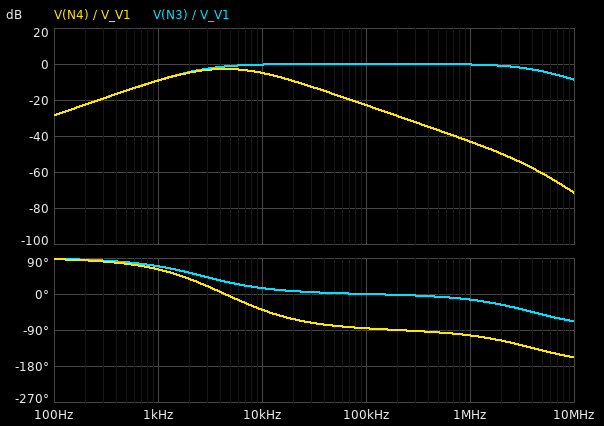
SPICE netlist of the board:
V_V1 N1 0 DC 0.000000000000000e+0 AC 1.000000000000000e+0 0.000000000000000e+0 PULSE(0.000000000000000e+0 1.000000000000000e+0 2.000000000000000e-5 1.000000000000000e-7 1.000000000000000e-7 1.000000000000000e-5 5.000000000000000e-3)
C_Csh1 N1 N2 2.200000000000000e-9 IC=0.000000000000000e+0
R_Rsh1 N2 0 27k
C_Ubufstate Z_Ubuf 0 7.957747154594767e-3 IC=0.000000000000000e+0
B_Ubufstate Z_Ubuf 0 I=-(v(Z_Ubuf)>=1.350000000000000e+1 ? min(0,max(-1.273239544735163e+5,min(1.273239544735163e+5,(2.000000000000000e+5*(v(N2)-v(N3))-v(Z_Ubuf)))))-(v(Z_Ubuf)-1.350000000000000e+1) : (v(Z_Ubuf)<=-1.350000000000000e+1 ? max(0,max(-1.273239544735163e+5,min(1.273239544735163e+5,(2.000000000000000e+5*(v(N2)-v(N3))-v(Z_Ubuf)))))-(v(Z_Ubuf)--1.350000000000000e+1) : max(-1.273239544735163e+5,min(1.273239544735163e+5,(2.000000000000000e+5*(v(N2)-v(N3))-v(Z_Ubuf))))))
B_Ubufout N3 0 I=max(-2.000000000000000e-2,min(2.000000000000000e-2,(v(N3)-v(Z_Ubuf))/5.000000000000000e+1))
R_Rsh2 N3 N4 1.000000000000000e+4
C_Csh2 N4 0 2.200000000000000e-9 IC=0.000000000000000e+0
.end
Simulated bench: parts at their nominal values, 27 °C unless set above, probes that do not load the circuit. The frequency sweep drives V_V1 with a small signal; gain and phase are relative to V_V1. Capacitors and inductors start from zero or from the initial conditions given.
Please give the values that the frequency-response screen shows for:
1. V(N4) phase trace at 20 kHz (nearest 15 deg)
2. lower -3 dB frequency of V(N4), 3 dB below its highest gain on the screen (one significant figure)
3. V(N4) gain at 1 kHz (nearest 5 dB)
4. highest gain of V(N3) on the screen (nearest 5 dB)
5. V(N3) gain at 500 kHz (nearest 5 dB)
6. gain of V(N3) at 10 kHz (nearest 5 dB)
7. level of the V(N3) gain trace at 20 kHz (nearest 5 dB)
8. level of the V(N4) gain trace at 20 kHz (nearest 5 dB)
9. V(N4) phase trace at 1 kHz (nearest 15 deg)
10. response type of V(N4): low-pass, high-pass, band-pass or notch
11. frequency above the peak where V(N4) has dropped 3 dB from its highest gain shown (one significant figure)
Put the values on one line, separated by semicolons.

-60 deg; 2 kHz; -10 dB; 0 dB; 0 dB; 0 dB; 0 dB; -10 dB; 60 deg; band-pass; 10 kHz
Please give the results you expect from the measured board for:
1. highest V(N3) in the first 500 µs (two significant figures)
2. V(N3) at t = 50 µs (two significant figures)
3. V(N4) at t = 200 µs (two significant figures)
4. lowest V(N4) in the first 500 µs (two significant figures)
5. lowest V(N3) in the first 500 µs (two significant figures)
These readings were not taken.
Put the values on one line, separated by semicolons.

1.0 V; -110 mV; -14 mV; -53 mV; -160 mV
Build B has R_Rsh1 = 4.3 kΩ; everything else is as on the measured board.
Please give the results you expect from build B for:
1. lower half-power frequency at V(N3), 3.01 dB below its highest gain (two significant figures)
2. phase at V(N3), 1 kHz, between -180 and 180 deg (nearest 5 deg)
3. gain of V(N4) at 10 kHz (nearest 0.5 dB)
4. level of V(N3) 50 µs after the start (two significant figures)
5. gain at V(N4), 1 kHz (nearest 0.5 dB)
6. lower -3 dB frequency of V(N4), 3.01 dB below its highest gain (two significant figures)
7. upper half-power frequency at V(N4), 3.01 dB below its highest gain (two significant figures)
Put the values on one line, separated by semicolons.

17 kHz; 85 deg; -10.5 dB; -81 mV; -24.5 dB; 4.3 kHz; 28 kHz
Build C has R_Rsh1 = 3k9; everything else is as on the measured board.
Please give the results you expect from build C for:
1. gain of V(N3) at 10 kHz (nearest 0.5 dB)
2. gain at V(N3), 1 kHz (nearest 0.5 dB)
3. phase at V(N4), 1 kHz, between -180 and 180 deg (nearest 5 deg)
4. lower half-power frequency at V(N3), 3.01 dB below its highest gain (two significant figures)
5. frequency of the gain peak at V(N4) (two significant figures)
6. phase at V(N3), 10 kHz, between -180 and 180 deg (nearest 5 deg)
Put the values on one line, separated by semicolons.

-6.5 dB; -25.5 dB; 80 deg; 18 kHz; 12 kHz; 60 deg
